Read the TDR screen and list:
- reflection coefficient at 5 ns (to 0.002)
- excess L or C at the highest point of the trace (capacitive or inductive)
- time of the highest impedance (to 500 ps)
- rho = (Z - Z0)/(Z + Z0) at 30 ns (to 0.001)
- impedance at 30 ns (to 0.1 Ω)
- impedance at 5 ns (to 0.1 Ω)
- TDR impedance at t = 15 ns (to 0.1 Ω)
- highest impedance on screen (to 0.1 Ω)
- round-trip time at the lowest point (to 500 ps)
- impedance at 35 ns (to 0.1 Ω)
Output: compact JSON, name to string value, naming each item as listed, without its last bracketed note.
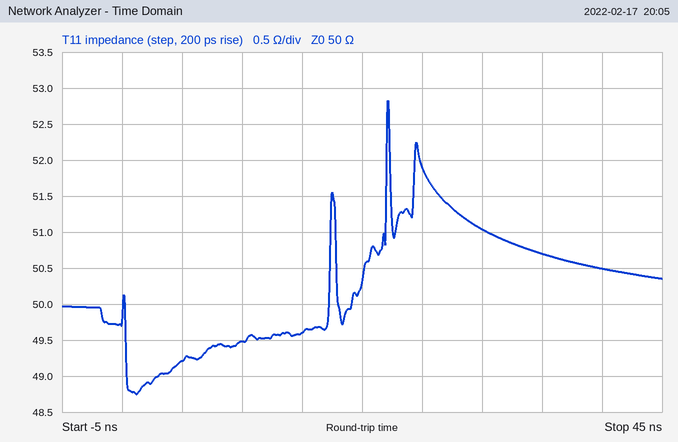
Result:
{"reflection coefficient at 5 ns": "-0.008", "excess L or C at the highest point of the trace": "inductive", "time of the highest impedance": "22.0 ns", "rho = (Z - Z0)/(Z + Z0) at 30 ns": "+0.010", "impedance at 30 ns": "51.0 Ω", "impedance at 5 ns": "49.2 Ω", "TDR impedance at t = 15 ns": "49.6 Ω", "highest impedance on screen": "52.8 Ω", "round-trip time at the lowest point": "1.0 ns", "impedance at 35 ns": "50.7 Ω"}
